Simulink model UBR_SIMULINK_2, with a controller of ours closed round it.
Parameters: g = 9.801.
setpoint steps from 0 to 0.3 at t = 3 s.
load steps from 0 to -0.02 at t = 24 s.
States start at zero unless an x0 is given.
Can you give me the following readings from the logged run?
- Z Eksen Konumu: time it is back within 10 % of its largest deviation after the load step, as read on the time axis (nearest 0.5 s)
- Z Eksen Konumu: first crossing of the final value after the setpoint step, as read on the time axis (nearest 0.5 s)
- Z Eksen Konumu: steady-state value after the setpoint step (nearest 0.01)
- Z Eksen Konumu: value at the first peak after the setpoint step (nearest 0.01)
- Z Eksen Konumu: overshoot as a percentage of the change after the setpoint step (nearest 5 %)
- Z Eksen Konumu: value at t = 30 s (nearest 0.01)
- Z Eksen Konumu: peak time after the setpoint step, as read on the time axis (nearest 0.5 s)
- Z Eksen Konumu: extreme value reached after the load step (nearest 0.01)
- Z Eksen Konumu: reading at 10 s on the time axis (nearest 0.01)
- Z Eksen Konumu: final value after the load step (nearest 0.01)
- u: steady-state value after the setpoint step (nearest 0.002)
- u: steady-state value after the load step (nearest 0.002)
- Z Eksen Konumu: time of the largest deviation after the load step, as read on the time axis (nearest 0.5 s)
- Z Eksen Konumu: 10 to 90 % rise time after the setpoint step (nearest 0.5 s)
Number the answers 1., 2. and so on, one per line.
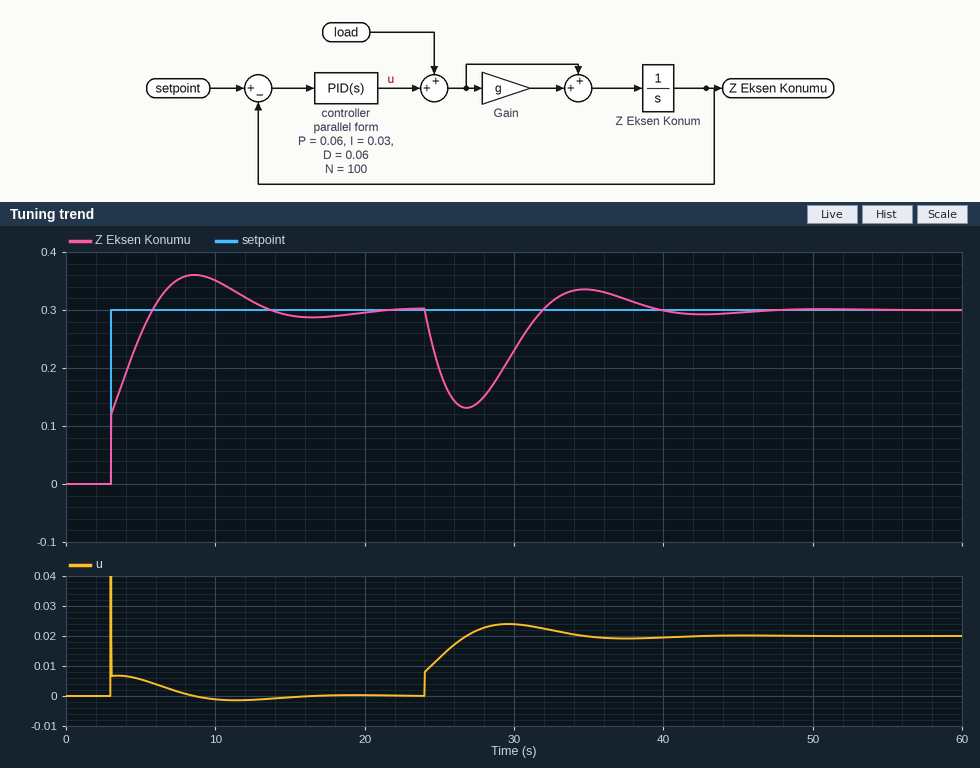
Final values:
1. 37.5 s
2. 6.0 s
3. 0.30
4. 0.36
5. 20 %
6. 0.23
7. 8.5 s
8. 0.13
9. 0.35
10. 0.30
11. 0.000
12. 0.020
13. 27.0 s
14. 2.0 s
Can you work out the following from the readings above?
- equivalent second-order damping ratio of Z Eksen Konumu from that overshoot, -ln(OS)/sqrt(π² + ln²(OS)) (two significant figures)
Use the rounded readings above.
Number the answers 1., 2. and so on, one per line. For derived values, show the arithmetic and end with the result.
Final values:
1. ln(0.2) = -1.609; 1.609 / sqrt(9.870 + 2.590) = 0.46
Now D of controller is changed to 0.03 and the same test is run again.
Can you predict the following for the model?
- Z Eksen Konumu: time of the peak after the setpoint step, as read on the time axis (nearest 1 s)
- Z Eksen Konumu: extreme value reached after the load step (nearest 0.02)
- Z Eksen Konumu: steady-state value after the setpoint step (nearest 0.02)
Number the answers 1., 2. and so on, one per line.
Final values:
1. 8 s
2. 0.12
3. 0.30
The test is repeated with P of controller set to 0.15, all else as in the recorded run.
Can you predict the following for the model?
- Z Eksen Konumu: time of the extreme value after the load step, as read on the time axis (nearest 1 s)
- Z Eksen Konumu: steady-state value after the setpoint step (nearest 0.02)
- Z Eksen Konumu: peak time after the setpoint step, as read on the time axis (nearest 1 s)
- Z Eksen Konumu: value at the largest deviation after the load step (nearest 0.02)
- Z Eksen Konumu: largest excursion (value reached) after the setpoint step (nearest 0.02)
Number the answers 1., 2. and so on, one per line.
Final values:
1. 26 s
2. 0.30
3. 7 s
4. 0.20
5. 0.32
